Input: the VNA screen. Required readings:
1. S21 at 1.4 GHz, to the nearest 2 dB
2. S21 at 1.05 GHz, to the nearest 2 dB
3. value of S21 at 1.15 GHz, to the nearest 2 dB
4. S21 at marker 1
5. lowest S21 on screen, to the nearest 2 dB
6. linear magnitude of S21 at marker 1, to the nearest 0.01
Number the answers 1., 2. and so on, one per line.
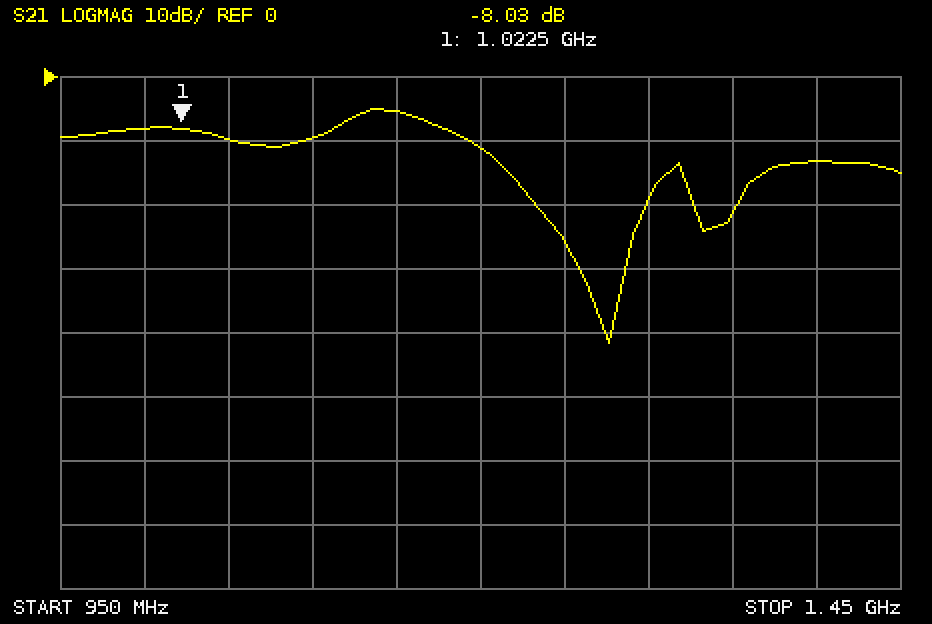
1. -14 dB
2. -10 dB
3. -6 dB
4. -8.03 dB
5. -42 dB
6. 0.40
